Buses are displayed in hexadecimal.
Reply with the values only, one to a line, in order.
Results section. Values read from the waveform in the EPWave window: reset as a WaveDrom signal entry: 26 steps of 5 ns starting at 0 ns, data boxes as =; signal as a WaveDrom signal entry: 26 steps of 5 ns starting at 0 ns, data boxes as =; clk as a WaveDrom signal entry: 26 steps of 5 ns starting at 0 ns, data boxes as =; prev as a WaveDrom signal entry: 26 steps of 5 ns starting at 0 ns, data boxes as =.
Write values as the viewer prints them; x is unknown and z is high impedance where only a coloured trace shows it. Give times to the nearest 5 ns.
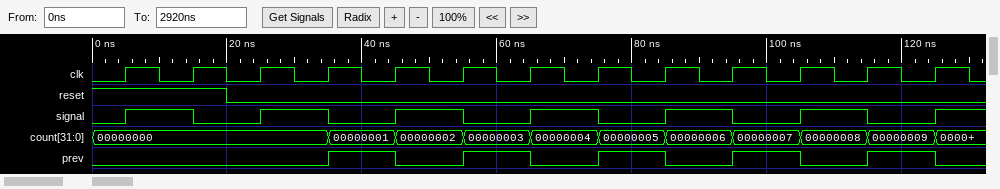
{name: 'reset', wave: '1...0.....................'}
{name: 'signal', wave: '01.0.1.0.1.0.1.0.1.0.1.0.1'}
{name: 'clk', wave: '01010101010101010101010101'}
{name: 'prev', wave: '0......1.0.1.0.1.0.1.0.1.0'}
